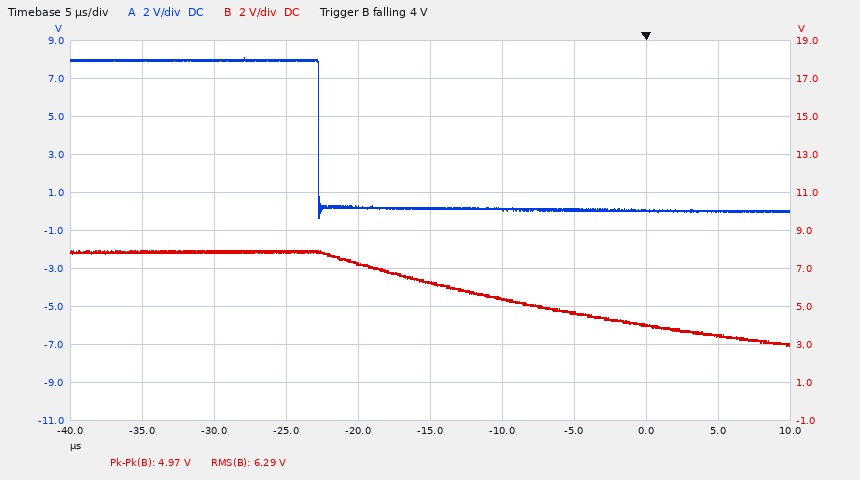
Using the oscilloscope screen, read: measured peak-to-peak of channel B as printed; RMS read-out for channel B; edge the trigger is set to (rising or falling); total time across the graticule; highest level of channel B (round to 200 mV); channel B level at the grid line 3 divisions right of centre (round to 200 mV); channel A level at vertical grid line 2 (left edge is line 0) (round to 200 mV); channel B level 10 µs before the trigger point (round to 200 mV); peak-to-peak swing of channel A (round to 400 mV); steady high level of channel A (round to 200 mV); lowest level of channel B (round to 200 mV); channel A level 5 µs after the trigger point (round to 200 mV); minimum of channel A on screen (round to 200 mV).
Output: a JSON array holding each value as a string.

["4.97 V", "6.29 V", "falling", "50 µs", "8.0 V", "4.0 V", "8.0 V", "5.4 V", "8.4 V", "8.0 V", "3.0 V", "0.0 V", "-400 mV"]
